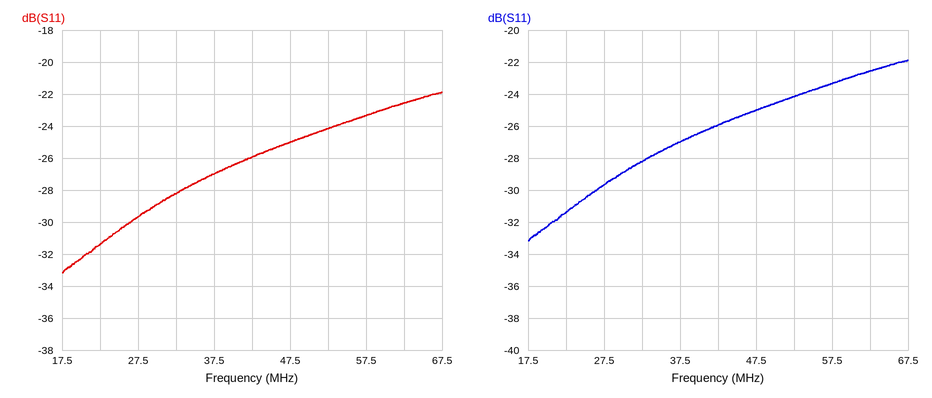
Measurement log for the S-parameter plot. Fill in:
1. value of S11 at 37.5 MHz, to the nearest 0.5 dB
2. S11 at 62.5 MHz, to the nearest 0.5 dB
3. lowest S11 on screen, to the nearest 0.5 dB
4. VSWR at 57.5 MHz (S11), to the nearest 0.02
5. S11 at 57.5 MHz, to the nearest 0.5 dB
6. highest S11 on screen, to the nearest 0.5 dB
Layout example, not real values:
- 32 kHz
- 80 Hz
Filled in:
- -27.0 dB
- -22.5 dB
- -33.0 dB
- 1.14
- -23.5 dB
- -22.0 dB
